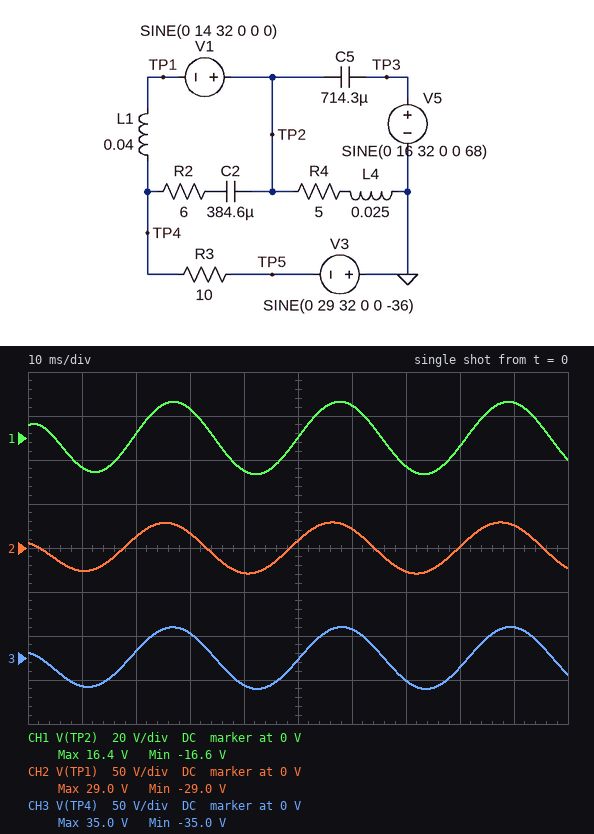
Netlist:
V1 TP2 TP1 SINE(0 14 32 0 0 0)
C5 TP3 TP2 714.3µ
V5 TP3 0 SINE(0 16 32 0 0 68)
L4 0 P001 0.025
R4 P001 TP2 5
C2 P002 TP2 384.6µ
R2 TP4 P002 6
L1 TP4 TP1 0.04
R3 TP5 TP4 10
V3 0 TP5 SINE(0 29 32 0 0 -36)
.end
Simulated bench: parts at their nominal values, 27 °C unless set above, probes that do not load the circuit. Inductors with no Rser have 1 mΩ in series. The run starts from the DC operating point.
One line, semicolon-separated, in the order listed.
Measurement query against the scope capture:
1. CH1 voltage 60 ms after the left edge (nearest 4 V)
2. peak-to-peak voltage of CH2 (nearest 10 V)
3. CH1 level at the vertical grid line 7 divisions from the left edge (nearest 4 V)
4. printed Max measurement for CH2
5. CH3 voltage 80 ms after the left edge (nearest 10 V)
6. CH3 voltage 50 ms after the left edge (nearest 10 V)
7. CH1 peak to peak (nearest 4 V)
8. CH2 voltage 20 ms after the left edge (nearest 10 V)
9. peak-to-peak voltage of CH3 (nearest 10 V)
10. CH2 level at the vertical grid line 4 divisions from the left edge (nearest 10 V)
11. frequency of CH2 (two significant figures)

16 V; 60 V; -12 V; 29.0 V; -10 V; 0 V; 32 V; 10 V; 70 V; -30 V; 32 Hz
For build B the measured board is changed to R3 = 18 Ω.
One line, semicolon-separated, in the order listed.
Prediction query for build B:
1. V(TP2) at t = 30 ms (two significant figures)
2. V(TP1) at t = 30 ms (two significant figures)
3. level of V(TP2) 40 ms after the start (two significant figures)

14 V; 18 V; -15 V
